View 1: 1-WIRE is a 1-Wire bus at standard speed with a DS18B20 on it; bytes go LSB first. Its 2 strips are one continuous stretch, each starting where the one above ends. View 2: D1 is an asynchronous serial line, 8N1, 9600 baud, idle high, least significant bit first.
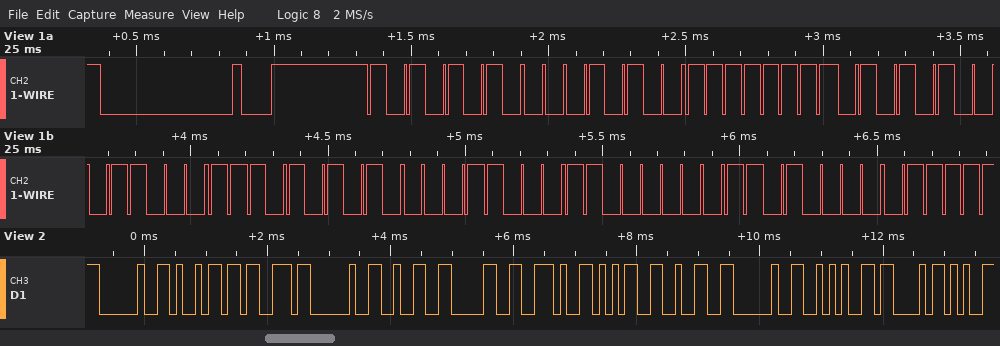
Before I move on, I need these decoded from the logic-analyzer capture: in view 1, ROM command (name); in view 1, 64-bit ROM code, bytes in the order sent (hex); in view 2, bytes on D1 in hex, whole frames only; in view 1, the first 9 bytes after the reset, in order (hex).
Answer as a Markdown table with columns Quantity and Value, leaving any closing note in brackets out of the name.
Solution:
| Quantity | Value |
|---|---|
| in view 1, ROM command | Match ROM |
| in view 1, 64-bit ROM code, bytes in the order sent | 28 FF 2A C6 55 18 03 0B |
| in view 2, bytes on D1 in hex, whole frames only | 0x20 0x69 0x73 0x20 0x32 0x30 0x2E 0x35 0x32 0x20 0x2A 0x43 |
| in view 1, the first 9 bytes after the reset, in order | 55 28 FF 2A C6 55 18 03 0B |
